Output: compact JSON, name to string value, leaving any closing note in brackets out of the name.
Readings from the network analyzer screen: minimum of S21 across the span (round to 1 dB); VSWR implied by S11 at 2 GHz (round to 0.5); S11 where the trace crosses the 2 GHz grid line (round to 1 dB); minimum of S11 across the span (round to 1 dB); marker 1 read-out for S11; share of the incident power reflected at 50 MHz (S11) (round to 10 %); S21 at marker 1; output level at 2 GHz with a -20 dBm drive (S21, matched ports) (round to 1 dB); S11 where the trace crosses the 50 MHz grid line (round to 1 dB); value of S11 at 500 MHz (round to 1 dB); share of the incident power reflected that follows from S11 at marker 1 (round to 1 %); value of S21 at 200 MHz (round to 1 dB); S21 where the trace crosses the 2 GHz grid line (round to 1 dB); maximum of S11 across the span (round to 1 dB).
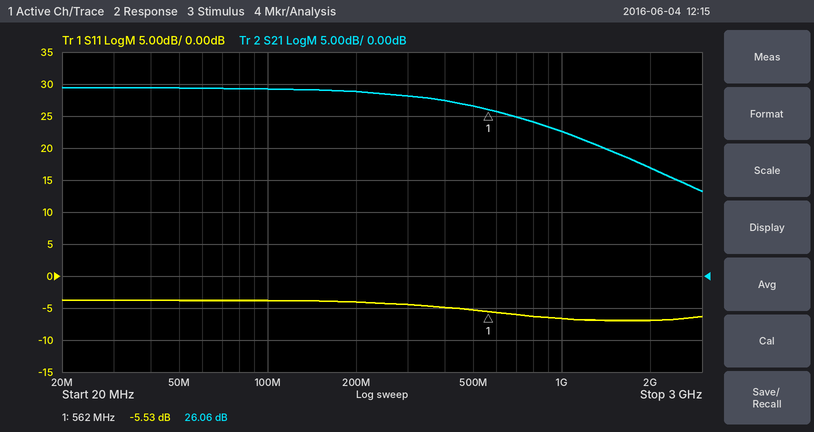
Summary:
{"minimum of S21 across the span": "13 dB", "VSWR implied by S11 at 2 GHz": "2.5", "S11 where the trace crosses the 2 GHz grid line": "-7 dB", "minimum of S11 across the span": "-7 dB", "marker 1 read-out for S11": "-5.53 dB", "share of the incident power reflected at 50 MHz (S11)": "40 %", "S21 at marker 1": "26.06 dB", "output level at 2 GHz with a -20 dBm drive (S21, matched ports)": "-3 dBm", "S11 where the trace crosses the 50 MHz grid line": "-4 dB", "value of S11 at 500 MHz": "-5 dB", "share of the incident power reflected that follows from S11 at marker 1": "28 %", "value of S21 at 200 MHz": "29 dB", "S21 where the trace crosses the 2 GHz grid line": "17 dB", "maximum of S11 across the span": "-4 dB"}
